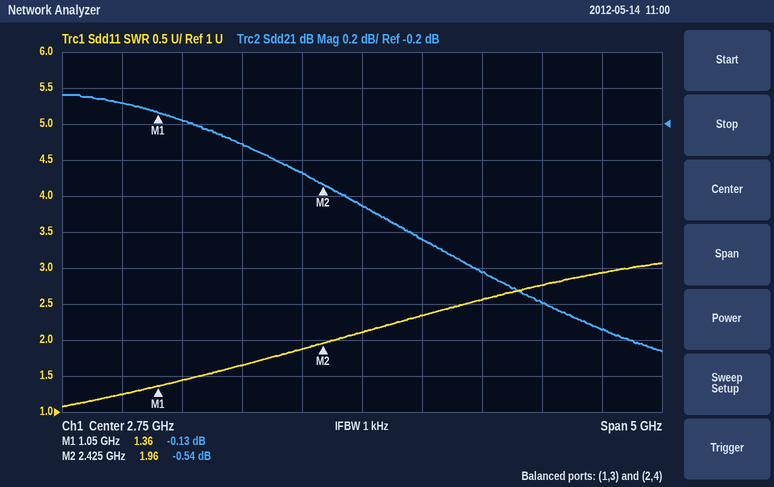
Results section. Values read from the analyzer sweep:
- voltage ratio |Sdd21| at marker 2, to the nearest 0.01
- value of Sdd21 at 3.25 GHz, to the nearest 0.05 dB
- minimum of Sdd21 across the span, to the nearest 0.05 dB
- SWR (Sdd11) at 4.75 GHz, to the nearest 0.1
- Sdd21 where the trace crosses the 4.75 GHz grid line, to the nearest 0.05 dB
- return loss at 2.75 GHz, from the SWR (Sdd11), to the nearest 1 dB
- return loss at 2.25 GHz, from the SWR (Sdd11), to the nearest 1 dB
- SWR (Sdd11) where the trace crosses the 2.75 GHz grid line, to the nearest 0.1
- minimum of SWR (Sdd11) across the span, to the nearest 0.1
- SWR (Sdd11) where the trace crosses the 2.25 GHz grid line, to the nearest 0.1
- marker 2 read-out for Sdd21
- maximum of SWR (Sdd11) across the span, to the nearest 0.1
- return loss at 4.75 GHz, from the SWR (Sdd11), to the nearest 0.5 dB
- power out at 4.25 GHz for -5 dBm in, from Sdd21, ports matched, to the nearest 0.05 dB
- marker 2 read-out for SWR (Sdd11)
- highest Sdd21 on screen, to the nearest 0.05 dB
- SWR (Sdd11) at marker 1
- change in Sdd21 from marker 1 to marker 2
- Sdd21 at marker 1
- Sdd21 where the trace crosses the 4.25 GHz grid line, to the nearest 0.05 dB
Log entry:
0.94
-0.85 dB
-1.45 dB
2.9
-1.35 dB
9 dB
10 dB
2.1
1.1
1.9
-0.54 dB
3.1
6.0 dB
-6.20 dBm
1.96
-0.05 dB
1.36
-0.41 dB
-0.13 dB
-1.20 dB
